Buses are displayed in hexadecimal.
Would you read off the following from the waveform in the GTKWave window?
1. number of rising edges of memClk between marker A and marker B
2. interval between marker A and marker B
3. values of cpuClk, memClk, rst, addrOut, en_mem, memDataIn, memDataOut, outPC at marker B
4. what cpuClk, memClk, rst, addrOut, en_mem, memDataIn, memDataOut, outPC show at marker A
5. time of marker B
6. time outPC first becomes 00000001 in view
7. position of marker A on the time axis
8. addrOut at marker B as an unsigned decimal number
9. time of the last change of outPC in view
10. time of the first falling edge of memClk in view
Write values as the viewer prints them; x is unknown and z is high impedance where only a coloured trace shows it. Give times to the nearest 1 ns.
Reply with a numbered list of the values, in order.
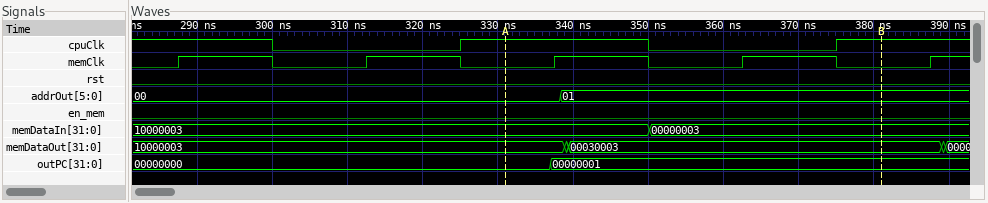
1. 2
2. 50 ns
3. cpuClk=1, memClk=0, rst=0, addrOut=01, en_mem=0, memDataIn=00000003, memDataOut=00030003, outPC=00000001
4. cpuClk=1, memClk=0, rst=0, addrOut=00, en_mem=0, memDataIn=10000003, memDataOut=10000003, outPC=00000000
5. 381 ns
6. 337 ns
7. 331 ns
8. 1
9. 337 ns
10. 300 ns
